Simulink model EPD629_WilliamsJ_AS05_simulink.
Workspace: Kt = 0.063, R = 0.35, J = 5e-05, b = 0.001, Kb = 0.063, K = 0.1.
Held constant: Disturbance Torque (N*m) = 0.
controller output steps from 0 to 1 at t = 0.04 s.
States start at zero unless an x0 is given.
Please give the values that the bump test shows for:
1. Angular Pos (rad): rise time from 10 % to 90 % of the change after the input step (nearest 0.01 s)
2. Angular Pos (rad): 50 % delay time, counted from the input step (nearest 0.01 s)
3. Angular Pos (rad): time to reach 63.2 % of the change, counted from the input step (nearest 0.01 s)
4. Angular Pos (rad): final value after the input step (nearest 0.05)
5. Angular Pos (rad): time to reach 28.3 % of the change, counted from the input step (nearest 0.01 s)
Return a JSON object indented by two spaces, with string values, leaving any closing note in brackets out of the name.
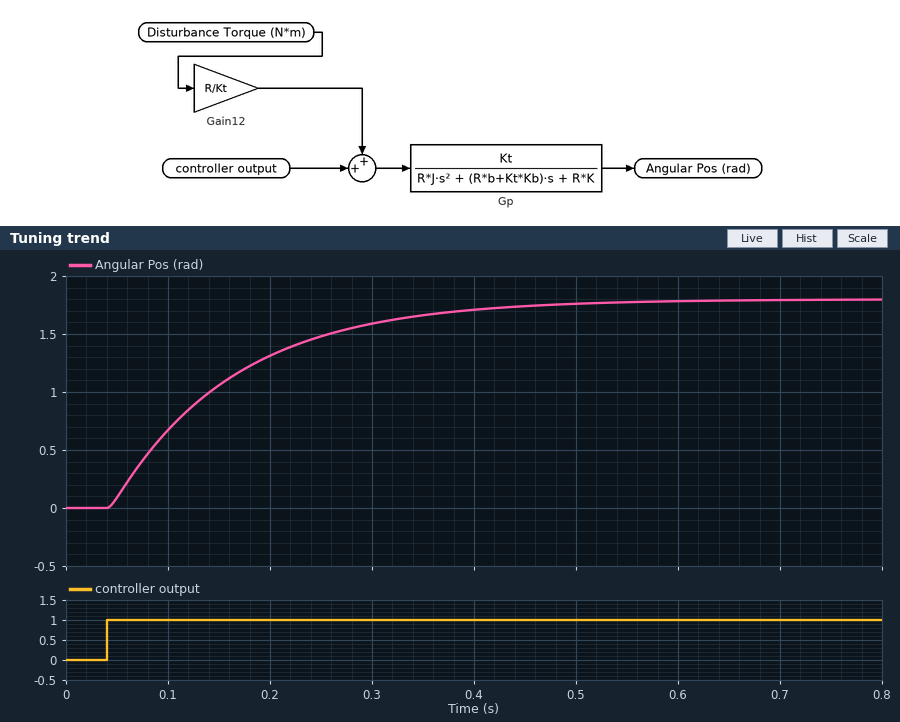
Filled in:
{
  "Angular Pos (rad): rise time from 10 % to 90 % of the change after the input step": "0.26 s",
  "Angular Pos (rad): 50 % delay time, counted from the input step": "0.09 s",
  "Angular Pos (rad): time to reach 63.2 % of the change, counted from the input step": "0.12 s",
  "Angular Pos (rad): final value after the input step": "1.80",
  "Angular Pos (rad): time to reach 28.3 % of the change, counted from the input step": "0.04 s"
}
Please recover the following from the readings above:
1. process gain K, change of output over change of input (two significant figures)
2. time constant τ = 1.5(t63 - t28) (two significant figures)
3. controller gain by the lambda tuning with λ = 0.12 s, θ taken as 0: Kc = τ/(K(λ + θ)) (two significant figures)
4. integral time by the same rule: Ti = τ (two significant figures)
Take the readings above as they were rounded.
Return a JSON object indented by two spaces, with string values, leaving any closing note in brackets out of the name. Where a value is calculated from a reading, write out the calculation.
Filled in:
{
  "process gain K, change of output over change of input": "(1.8 - 0) / 1 = 1.8",
  "time constant τ = 1.5(t63 - t28)": "1.5 × (0.12 - 0.04) = 0.12 s",
  "controller gain by the lambda tuning with λ = 0.12 s, θ taken as 0: Kc = τ/(K(λ + θ))": "0.12 / (1.8 × (0.12 + 0)) = 0.56",
  "integral time by the same rule: Ti = τ": "0.12 s"
}
